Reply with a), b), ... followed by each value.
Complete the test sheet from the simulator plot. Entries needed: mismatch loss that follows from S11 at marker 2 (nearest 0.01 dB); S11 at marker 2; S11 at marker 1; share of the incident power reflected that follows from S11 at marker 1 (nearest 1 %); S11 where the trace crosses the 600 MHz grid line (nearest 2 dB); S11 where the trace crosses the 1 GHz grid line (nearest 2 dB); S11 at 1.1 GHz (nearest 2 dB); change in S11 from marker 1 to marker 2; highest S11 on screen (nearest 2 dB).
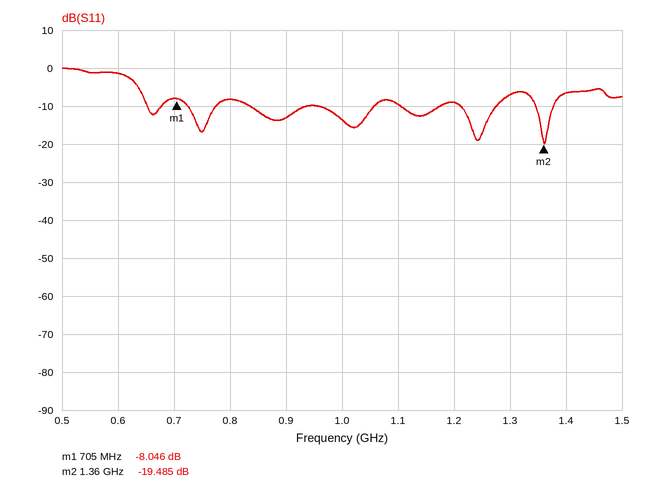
a) 0.05 dB
b) -19.485 dB
c) -8.046 dB
d) 16 %
e) -2 dB
f) -14 dB
g) -10 dB
h) -11.439 dB
i) 0 dB
